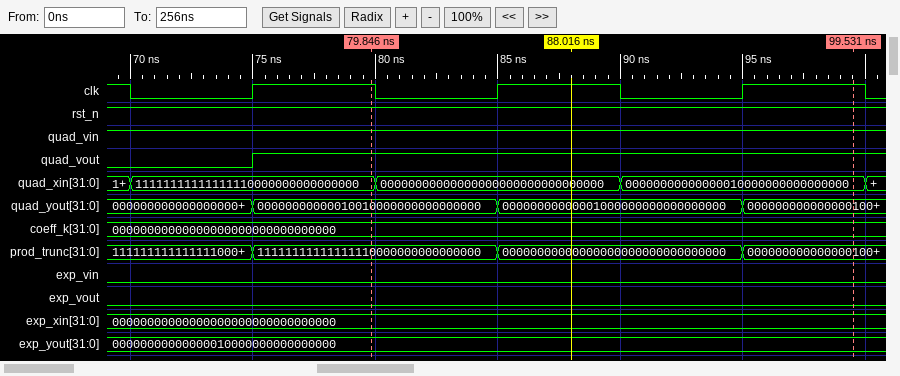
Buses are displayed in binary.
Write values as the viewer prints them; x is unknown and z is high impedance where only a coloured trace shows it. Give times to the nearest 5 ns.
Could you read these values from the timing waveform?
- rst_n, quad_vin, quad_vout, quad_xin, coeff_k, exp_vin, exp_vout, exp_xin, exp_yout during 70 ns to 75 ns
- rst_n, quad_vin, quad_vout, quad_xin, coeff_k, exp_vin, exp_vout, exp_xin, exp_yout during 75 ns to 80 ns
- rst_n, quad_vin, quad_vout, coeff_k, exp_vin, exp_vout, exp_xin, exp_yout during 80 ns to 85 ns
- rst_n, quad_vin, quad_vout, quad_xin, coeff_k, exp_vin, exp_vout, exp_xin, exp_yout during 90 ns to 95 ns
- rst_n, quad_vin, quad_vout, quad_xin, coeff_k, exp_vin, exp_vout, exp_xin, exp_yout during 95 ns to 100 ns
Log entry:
rst_n=1, quad_vin=1, quad_vout=0, quad_xin=11111111111111110000000000000000, coeff_k=00000000000000000000000000000000, exp_vin=0, exp_vout=0, exp_xin=00000000000000000000000000000000, exp_yout=00000000000000010000000000000000
rst_n=1, quad_vin=1, quad_vout=1, quad_xin=11111111111111110000000000000000, coeff_k=00000000000000000000000000000000, exp_vin=0, exp_vout=0, exp_xin=00000000000000000000000000000000, exp_yout=00000000000000010000000000000000
rst_n=1, quad_vin=1, quad_vout=1, coeff_k=00000000000000000000000000000000, exp_vin=0, exp_vout=0, exp_xin=00000000000000000000000000000000, exp_yout=00000000000000010000000000000000
rst_n=1, quad_vin=1, quad_vout=1, quad_xin=00000000000000010000000000000000, coeff_k=00000000000000000000000000000000, exp_vin=0, exp_vout=0, exp_xin=00000000000000000000000000000000, exp_yout=00000000000000010000000000000000
rst_n=1, quad_vin=1, quad_vout=1, quad_xin=00000000000000010000000000000000, coeff_k=00000000000000000000000000000000, exp_vin=0, exp_vout=0, exp_xin=00000000000000000000000000000000, exp_yout=00000000000000010000000000000000
